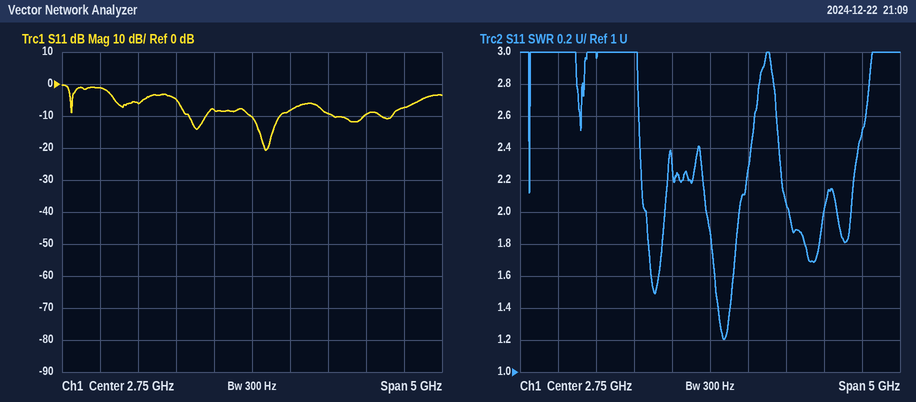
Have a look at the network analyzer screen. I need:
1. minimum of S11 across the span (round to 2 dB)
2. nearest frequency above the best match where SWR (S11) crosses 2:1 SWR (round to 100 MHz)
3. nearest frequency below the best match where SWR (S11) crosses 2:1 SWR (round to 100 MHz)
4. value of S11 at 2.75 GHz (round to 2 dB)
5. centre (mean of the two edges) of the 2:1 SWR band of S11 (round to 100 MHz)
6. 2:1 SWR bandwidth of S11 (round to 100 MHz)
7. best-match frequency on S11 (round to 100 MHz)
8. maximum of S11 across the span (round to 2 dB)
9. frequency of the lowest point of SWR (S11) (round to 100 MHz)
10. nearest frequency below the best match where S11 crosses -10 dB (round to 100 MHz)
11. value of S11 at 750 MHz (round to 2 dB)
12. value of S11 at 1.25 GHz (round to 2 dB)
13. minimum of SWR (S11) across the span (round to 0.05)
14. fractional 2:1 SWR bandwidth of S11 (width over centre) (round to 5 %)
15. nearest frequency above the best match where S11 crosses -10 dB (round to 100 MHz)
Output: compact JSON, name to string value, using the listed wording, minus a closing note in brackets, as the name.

{"minimum of S11 across the span": "-20 dB", "nearest frequency above the best match where SWR (S11) crosses 2:1 SWR": "3.1 GHz", "nearest frequency below the best match where SWR (S11) crosses 2:1 SWR": "2.7 GHz", "value of S11 at 2.75 GHz": "-10 dB", "centre (mean of the two edges) of the 2:1 SWR band of S11": "2.9 GHz", "2:1 SWR bandwidth of S11": "400 MHz", "best-match frequency on S11": "2.9 GHz", "maximum of S11 across the span": "0 dB", "frequency of the lowest point of SWR (S11)": "2.9 GHz", "nearest frequency below the best match where S11 crosses -10 dB": "2.7 GHz", "value of S11 at 750 MHz": "-2 dB", "value of S11 at 1.25 GHz": "-6 dB", "minimum of SWR (S11) across the span": "1.20", "fractional 2:1 SWR bandwidth of S11 (width over centre)": "15 %", "nearest frequency above the best match where S11 crosses -10 dB": "3.1 GHz"}
